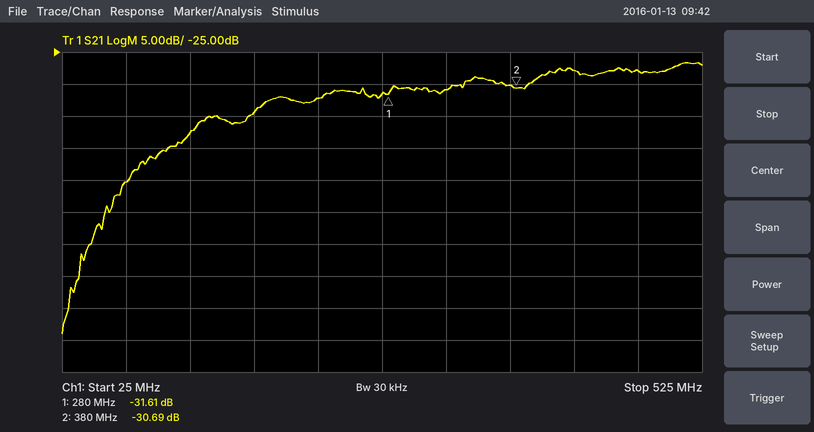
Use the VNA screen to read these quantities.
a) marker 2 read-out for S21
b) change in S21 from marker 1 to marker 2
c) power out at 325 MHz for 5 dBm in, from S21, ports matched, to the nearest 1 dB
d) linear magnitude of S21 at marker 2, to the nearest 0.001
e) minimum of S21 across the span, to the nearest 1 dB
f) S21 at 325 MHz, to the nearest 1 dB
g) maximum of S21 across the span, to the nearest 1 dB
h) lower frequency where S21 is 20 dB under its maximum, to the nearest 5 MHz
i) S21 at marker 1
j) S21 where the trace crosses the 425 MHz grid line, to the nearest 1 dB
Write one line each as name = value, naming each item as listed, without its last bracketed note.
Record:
marker 2 read-out for S21 = -30.69 dB
change in S21 from marker 1 to marker 2 = 0.92 dB
power out at 325 MHz for 5 dBm in, from S21, ports matched, to the nearest 1 dB = -26 dBm
linear magnitude of S21 at marker 2, to the nearest 0.001 = 0.029
minimum of S21 across the span, to the nearest 1 dB = -69 dB
S21 at 325 MHz, to the nearest 1 dB = -31 dB
maximum of S21 across the span, to the nearest 1 dB = -27 dB
lower frequency where S21 is 20 dB under its maximum, to the nearest 5 MHz = 70 MHz
S21 at marker 1 = -31.61 dB
S21 where the trace crosses the 425 MHz grid line, to the nearest 1 dB = -28 dB
